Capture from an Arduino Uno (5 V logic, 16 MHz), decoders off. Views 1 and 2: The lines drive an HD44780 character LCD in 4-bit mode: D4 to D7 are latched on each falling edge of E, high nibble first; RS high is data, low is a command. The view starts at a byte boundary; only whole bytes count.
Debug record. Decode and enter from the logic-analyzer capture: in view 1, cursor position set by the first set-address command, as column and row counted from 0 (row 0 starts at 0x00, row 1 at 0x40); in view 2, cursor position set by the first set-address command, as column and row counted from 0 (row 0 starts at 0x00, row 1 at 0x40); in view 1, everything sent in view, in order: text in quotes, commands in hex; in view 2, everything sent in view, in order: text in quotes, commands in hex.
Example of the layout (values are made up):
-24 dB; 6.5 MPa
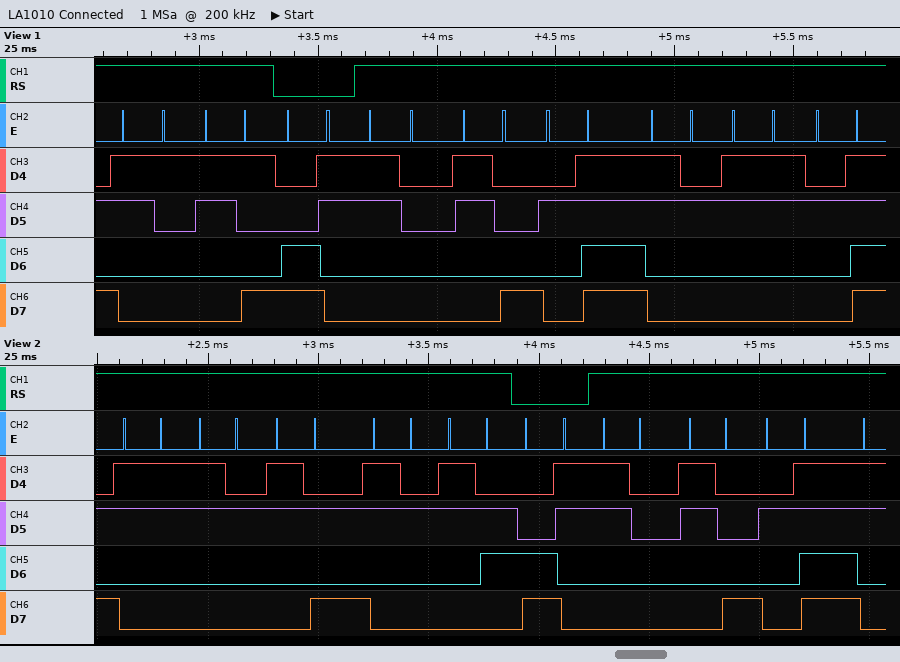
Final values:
column 3, row 1; column 3, row 1; "19" 0xC3 "08/23/"; "32:26" 0xC3 "08/"
